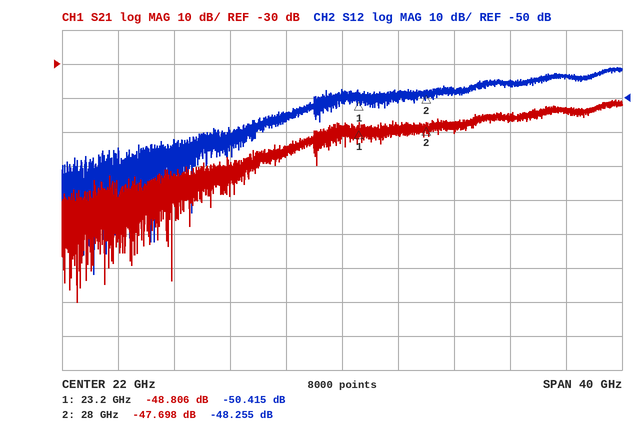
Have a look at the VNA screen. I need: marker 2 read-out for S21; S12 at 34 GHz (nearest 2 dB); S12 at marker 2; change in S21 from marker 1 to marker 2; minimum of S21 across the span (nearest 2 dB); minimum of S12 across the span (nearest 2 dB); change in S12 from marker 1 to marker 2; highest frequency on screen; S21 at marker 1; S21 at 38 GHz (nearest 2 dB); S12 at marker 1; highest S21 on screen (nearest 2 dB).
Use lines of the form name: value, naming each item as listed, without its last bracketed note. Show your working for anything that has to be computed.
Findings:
marker 2 read-out for S21: -47.698 dB
S12 at 34 GHz: -46 dB
S12 at marker 2: -48.255 dB
change in S21 from marker 1 to marker 2: -47.698 − (-48.806) = 1.108 dB
minimum of S21 across the span: -100 dB
minimum of S12 across the span: -102 dB
change in S12 from marker 1 to marker 2: -48.255 − (-50.415) = 2.160 dB
highest frequency on screen: 42 GHz
S21 at marker 1: -48.806 dB
S21 at 38 GHz: -44 dB
S12 at marker 1: -50.415 dB
highest S21 on screen: -40 dB
